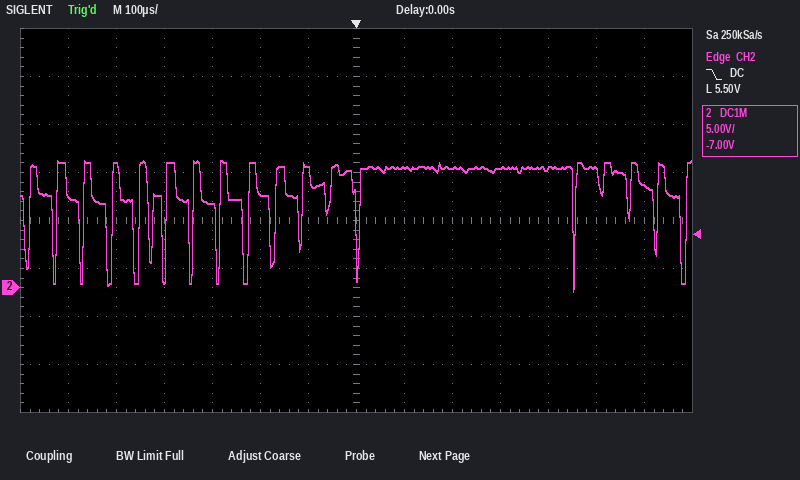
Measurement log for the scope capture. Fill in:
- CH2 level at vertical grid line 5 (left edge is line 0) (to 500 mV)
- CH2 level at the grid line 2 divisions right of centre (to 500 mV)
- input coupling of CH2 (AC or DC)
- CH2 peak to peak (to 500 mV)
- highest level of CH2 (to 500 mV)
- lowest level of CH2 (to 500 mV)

10.0 V
12.5 V
DC
13.5 V
13.0 V
-500 mV
